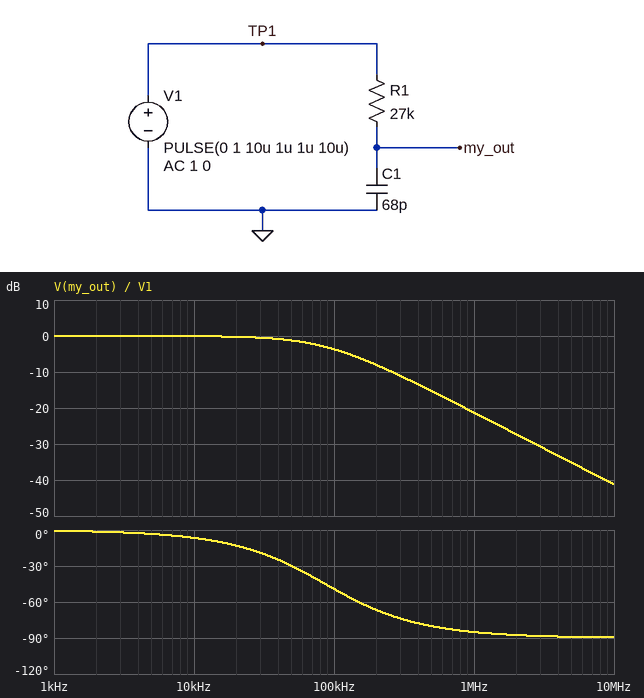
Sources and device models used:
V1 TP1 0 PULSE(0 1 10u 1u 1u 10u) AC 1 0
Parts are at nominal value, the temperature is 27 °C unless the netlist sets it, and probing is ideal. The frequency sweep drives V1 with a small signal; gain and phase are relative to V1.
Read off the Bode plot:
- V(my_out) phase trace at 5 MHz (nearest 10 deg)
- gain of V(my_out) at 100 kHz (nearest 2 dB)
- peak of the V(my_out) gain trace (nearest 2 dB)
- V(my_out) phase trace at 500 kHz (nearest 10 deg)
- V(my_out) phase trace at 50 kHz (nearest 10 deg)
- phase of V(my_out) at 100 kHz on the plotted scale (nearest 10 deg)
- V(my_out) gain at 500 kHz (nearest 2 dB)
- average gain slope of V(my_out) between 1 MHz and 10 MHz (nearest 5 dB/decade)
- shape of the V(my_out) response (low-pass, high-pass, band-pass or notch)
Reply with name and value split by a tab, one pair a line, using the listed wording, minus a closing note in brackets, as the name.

V(my_out) phase trace at 5 MHz	-90 deg
gain of V(my_out) at 100 kHz	-4 dB
peak of the V(my_out) gain trace	0 dB
V(my_out) phase trace at 500 kHz	-80 deg
V(my_out) phase trace at 50 kHz	-30 deg
phase of V(my_out) at 100 kHz on the plotted scale	-50 deg
V(my_out) gain at 500 kHz	-16 dB
average gain slope of V(my_out) between 1 MHz and 10 MHz	-20 dB/decade
shape of the V(my_out) response	low-pass
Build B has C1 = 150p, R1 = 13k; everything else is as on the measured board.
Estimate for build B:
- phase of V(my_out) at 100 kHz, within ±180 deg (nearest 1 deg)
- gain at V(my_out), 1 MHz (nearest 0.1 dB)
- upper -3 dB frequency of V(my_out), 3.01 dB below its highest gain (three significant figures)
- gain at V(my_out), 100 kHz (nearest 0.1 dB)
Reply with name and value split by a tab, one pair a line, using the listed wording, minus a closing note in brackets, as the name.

phase of V(my_out) at 100 kHz, within ±180 deg	-51 deg
gain at V(my_out), 1 MHz	-21.8 dB
upper -3 dB frequency of V(my_out), 3.01 dB below its highest gain	81.6 kHz
gain at V(my_out), 100 kHz	-4.0 dB
